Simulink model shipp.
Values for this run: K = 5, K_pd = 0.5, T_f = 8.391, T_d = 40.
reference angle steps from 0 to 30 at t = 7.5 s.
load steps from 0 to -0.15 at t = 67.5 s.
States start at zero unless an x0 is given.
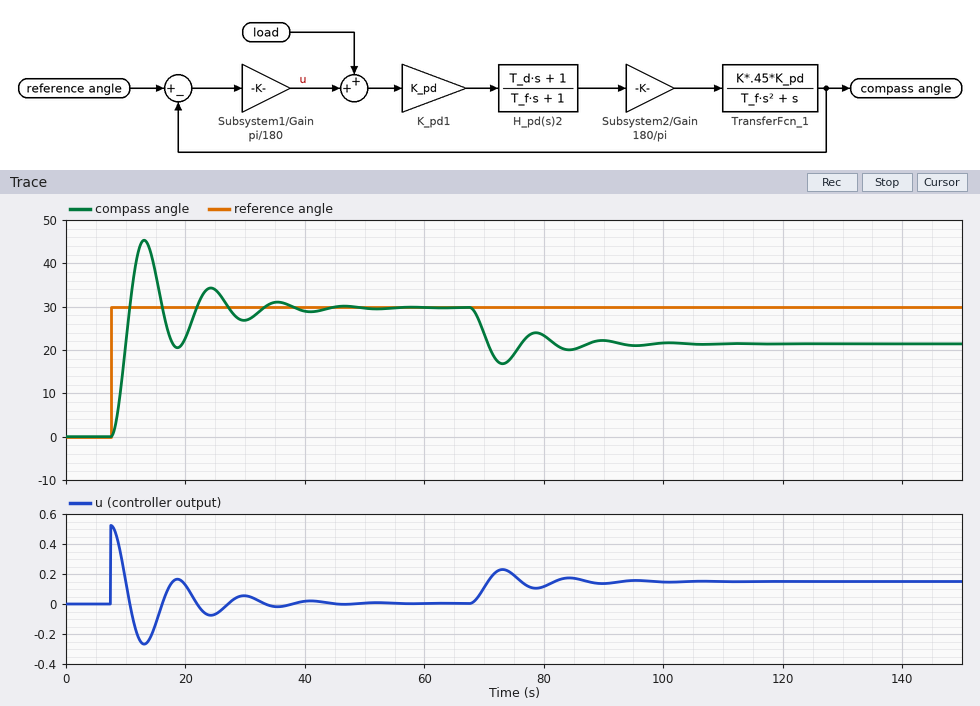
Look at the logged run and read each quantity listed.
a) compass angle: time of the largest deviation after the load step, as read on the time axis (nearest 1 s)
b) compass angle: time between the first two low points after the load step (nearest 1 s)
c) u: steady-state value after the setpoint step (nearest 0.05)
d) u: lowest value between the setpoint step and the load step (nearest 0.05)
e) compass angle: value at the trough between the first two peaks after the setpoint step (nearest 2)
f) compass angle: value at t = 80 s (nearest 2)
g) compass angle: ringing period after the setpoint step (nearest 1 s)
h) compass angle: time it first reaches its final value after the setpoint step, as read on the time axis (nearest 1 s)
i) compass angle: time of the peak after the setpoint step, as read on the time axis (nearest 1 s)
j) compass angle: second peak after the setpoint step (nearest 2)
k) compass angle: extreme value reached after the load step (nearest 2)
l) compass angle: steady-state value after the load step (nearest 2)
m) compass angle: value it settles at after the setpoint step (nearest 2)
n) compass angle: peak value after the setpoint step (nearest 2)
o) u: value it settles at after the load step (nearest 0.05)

73 s
11 s
0.00
-0.25
20
24
11 s
11 s
13 s
34
16
22
30
46
0.15
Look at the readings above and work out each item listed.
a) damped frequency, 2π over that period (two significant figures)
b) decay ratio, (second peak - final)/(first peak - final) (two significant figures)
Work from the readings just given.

0.57 rad/s
0.25
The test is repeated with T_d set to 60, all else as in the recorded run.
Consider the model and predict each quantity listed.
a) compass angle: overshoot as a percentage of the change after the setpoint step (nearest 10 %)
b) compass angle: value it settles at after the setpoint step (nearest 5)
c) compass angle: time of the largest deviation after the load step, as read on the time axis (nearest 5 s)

60 %
30
70 s
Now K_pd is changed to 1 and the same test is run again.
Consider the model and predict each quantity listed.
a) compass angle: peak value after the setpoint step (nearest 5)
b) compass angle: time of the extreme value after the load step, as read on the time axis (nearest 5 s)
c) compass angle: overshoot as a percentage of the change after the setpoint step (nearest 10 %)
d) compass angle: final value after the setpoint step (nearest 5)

50
70 s
70 %
30
